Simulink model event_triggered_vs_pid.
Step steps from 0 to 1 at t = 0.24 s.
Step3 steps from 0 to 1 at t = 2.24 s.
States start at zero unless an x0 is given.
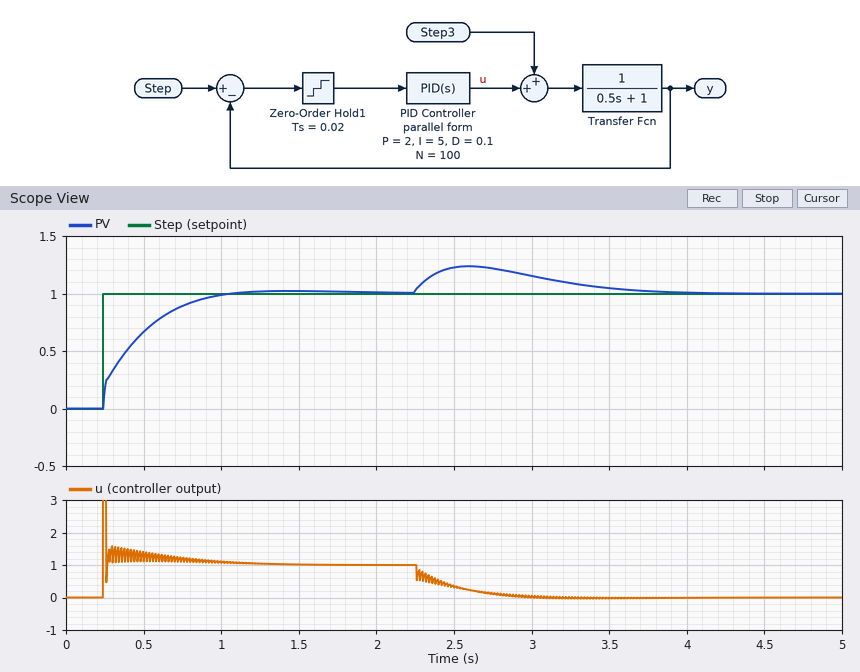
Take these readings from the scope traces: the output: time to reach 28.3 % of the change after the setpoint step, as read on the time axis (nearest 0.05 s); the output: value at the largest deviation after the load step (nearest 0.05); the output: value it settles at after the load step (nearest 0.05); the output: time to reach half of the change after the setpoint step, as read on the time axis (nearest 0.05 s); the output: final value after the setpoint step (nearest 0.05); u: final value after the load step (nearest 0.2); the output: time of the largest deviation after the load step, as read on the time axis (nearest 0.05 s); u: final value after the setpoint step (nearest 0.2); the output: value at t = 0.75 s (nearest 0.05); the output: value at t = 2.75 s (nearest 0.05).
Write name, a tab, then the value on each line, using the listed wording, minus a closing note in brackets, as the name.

the output: time to reach 28.3 % of the change after the setpoint step, as read on the time axis	0.30 s
the output: value at the largest deviation after the load step	1.25
the output: value it settles at after the load step	1.00
the output: time to reach half of the change after the setpoint step, as read on the time axis	0.40 s
the output: final value after the setpoint step	1.00
u: final value after the load step	0.0
the output: time of the largest deviation after the load step, as read on the time axis	2.60 s
u: final value after the setpoint step	1.0
the output: value at t = 0.75 s	0.90
the output: value at t = 2.75 s	1.20
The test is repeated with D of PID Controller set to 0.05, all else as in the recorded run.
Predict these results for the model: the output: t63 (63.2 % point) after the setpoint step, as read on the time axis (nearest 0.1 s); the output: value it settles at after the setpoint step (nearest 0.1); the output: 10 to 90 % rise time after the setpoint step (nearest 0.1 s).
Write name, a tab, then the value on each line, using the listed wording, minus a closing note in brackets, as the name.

the output: t63 (63.2 % point) after the setpoint step, as read on the time axis	0.5 s
the output: value it settles at after the setpoint step	1.0
the output: 10 to 90 % rise time after the setpoint step	0.5 s
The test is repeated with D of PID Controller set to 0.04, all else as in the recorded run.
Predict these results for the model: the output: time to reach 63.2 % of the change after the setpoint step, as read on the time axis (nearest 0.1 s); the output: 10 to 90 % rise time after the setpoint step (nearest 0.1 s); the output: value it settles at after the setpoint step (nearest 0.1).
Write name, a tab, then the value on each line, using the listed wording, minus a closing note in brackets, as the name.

the output: time to reach 63.2 % of the change after the setpoint step, as read on the time axis	0.5 s
the output: 10 to 90 % rise time after the setpoint step	0.5 s
the output: value it settles at after the setpoint step	1.0
